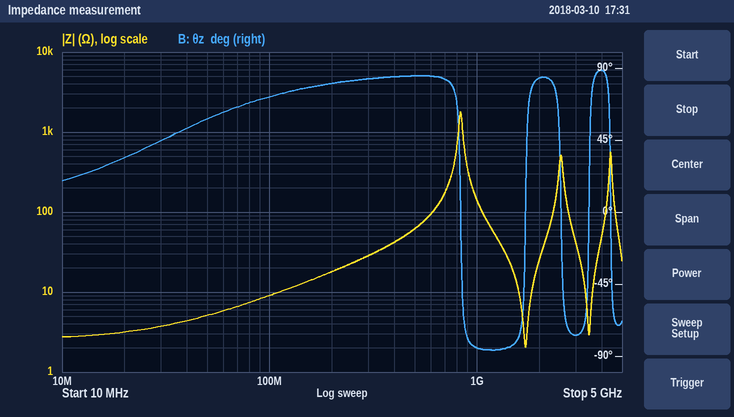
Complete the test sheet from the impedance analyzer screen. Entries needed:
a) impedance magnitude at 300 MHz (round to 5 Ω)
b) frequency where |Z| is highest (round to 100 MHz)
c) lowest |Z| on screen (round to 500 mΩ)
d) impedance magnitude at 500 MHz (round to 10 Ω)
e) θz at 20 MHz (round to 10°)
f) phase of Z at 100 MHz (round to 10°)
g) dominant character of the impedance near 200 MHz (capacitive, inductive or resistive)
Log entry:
30 Ω
800 MHz
2.0 Ω
60 Ω
30°
70°
inductive
